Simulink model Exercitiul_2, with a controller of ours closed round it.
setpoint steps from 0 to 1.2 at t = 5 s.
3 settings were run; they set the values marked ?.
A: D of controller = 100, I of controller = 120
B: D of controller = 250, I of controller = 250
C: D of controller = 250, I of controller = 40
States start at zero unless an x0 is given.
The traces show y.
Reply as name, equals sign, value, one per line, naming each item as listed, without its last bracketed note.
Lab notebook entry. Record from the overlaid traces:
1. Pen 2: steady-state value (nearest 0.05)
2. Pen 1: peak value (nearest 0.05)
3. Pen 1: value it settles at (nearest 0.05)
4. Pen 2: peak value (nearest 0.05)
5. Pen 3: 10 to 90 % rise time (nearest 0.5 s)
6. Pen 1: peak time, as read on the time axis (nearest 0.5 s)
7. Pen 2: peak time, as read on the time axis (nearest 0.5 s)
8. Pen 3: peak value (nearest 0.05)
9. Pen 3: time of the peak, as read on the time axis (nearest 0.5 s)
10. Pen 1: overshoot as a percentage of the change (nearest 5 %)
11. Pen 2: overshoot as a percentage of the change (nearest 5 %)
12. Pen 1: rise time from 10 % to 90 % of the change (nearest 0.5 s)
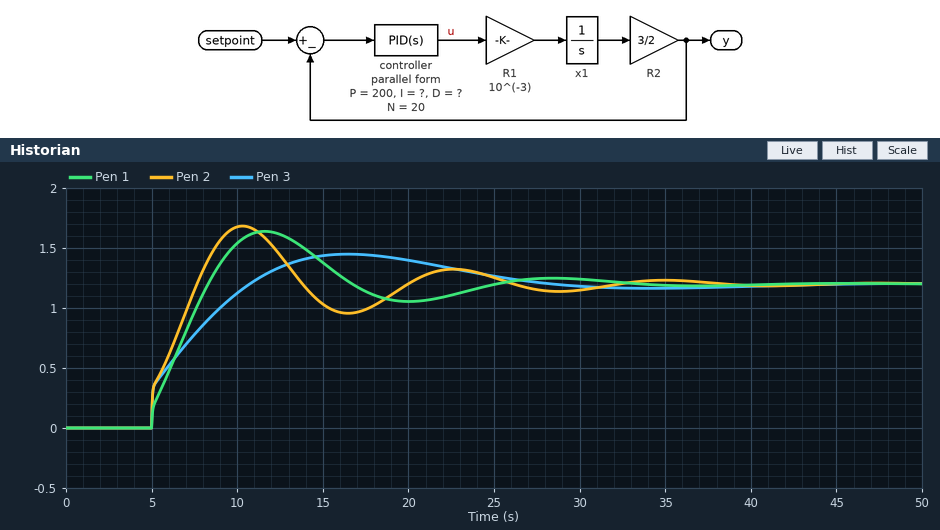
Pen 2: steady-state value = 1.20
Pen 1: peak value = 1.65
Pen 1: value it settles at = 1.20
Pen 2: peak value = 1.70
Pen 3: 10 to 90 % rise time = 4.5 s
Pen 1: peak time, as read on the time axis = 11.5 s
Pen 2: peak time, as read on the time axis = 10.5 s
Pen 3: peak value = 1.45
Pen 3: time of the peak, as read on the time axis = 16.5 s
Pen 1: overshoot as a percentage of the change = 35 %
Pen 2: overshoot as a percentage of the change = 40 %
Pen 1: rise time from 10 % to 90 % of the change = 3.0 s
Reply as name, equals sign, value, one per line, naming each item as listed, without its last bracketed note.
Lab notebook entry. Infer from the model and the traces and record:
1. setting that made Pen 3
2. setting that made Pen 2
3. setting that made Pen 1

setting that made Pen 3 = C
setting that made Pen 2 = B
setting that made Pen 1 = A
